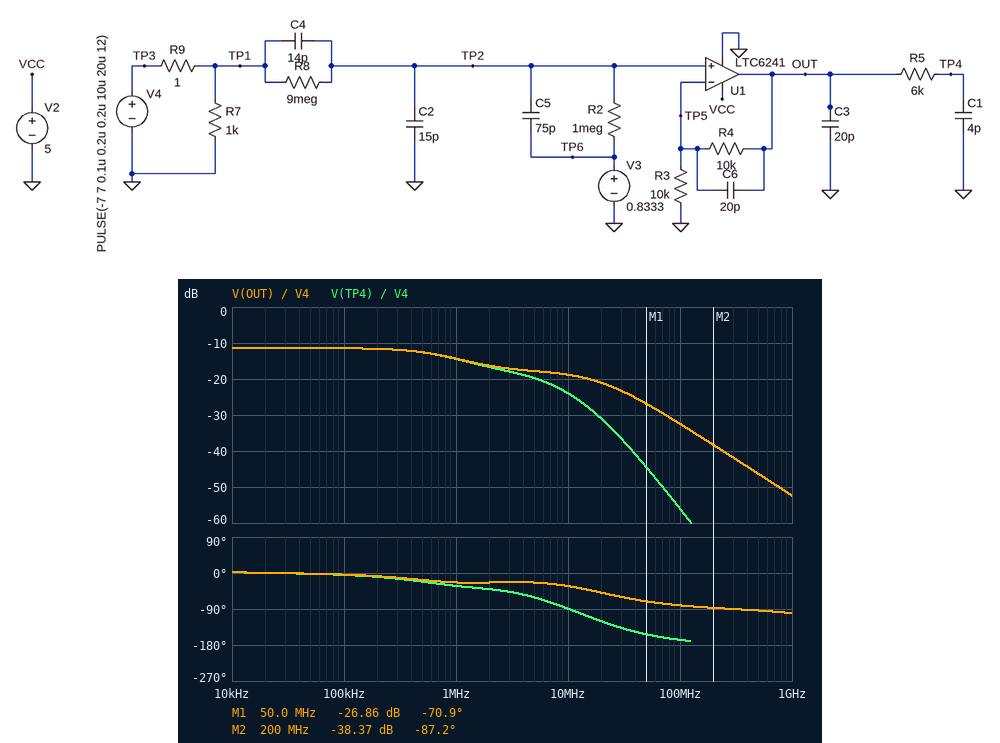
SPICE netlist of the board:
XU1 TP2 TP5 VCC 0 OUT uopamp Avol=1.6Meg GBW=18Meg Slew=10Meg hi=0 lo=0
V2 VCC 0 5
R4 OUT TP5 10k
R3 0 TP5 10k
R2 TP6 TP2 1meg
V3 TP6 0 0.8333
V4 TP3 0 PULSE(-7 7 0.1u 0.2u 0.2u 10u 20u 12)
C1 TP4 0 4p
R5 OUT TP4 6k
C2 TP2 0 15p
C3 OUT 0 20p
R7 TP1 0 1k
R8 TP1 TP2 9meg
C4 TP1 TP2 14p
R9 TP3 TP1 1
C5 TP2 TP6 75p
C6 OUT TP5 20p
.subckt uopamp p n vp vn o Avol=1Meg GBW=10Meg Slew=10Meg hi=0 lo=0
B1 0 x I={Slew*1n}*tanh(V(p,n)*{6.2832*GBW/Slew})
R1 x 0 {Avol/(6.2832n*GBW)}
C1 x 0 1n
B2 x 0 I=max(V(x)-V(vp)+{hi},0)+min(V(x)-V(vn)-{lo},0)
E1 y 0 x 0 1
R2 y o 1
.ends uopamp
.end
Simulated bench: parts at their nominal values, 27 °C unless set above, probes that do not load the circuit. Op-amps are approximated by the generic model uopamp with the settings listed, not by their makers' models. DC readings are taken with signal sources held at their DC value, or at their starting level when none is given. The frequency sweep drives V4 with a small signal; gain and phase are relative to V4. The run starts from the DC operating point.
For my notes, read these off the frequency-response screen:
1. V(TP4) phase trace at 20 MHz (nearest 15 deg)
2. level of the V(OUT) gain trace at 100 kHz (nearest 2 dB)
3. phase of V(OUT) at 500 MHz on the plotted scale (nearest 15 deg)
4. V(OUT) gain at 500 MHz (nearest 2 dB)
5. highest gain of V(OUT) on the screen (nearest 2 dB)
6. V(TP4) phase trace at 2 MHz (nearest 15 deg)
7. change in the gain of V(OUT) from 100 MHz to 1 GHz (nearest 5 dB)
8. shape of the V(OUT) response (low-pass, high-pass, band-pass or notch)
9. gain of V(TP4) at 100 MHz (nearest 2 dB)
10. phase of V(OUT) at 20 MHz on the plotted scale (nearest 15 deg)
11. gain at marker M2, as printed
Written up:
-120 deg
-12 dB
-90 deg
-46 dB
-12 dB
-45 deg
-20 dB
low-pass
-56 dB
-45 deg
-38.37 dB
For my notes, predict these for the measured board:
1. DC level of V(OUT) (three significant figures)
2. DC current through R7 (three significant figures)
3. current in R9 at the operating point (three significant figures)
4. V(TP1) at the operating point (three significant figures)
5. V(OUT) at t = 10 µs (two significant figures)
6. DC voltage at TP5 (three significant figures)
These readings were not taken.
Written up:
101 mV
6.99 mA
6.99 mA
-6.99 V
3.8 V
50.7 mV
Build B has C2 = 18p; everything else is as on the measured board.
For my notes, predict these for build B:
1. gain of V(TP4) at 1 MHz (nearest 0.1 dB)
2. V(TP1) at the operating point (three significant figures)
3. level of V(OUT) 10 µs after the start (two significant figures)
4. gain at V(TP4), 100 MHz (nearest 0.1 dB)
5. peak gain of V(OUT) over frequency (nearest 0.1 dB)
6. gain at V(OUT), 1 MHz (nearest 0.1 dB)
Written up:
-14.7 dB
-6.99 V
3.7 V
-56.3 dB
-11.7 dB
-14.6 dB
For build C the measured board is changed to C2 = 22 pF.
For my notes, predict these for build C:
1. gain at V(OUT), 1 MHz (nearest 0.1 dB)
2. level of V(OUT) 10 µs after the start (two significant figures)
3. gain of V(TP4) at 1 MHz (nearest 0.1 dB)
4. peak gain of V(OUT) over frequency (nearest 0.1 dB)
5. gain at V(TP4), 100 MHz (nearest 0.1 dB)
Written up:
-14.9 dB
3.6 V
-15.0 dB
-12.0 dB
-56.6 dB
